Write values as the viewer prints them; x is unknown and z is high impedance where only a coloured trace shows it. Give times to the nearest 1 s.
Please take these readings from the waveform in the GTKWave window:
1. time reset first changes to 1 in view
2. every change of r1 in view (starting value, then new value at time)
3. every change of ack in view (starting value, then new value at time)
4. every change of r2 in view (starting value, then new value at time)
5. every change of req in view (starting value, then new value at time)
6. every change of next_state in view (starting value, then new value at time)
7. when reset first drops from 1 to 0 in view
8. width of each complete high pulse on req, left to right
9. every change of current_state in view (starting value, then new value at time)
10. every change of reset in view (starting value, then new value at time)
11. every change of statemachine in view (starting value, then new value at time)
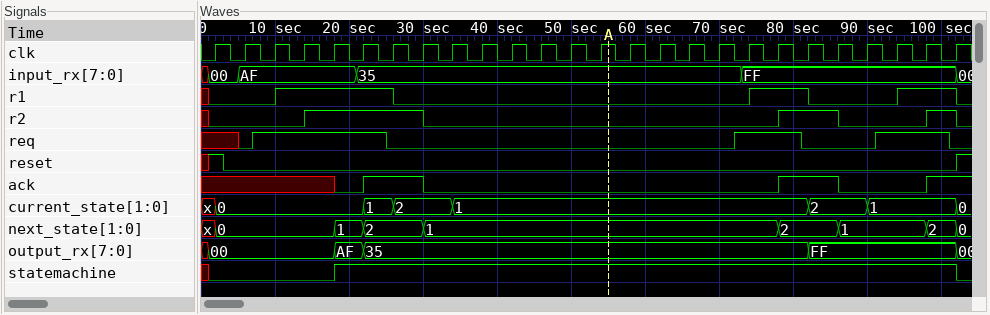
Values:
1 s
x, 0 at 1 s, 1 at 10 s, 0 at 26 s, 1 at 74 s, 0 at 82 s, 1 at 94 s, 0 at 102 s
x, 0 at 18 s, 1 at 22 s, 0 at 30 s, 1 at 78 s, 0 at 86 s, 1 at 98 s
x, 0 at 1 s, 1 at 14 s, 0 at 30 s, 1 at 78 s, 0 at 86 s, 1 at 98 s, 0 at 102 s
x, 0 at 5 s, 1 at 7 s, 0 at 25 s, 1 at 72 s, 0 at 81 s, 1 at 91 s, 0 at 101 s
x, 0 at 2 s, 1 at 18 s, 2 at 22 s, 1 at 30 s, 2 at 78 s, 1 at 86 s, 2 at 98 s, 0 at 102 s
3 s
18 s, 9 s, 10 s
x, 0 at 2 s, 1 at 22 s, 2 at 26 s, 1 at 34 s, 2 at 82 s, 1 at 90 s, 0 at 102 s
x, 1 at 1 s, 0 at 3 s, 1 at 102 s
x, 0 at 1 s, 1 at 18 s, 0 at 102 s
